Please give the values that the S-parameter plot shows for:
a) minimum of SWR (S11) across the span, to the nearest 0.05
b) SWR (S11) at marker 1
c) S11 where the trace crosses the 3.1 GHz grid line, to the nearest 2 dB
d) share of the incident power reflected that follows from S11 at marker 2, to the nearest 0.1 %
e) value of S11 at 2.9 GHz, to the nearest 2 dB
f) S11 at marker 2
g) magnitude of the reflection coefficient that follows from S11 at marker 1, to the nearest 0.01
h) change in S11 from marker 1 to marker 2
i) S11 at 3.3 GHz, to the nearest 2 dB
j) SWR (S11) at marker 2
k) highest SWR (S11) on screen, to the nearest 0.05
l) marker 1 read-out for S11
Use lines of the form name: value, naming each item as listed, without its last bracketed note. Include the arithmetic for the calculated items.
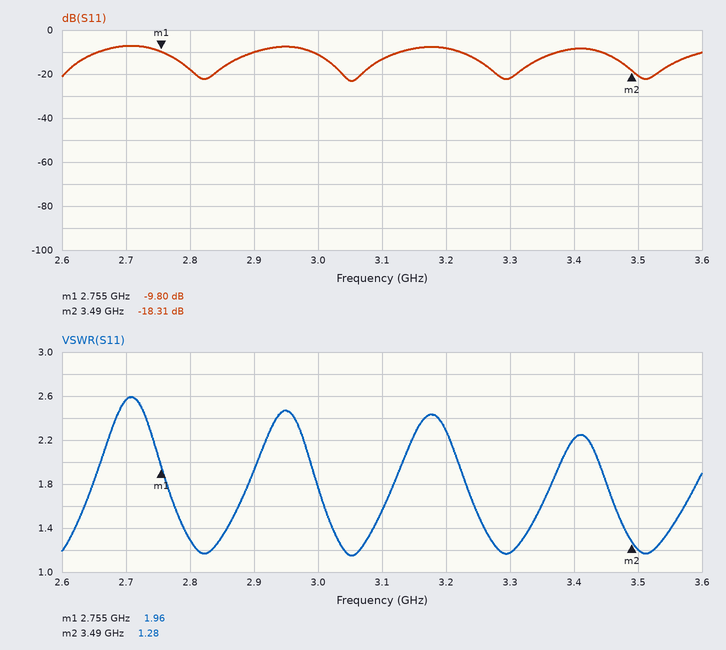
minimum of SWR (S11) across the span, to the nearest 0.05: 1.15
SWR (S11) at marker 1: 1.96
S11 where the trace crosses the 3.1 GHz grid line, to the nearest 2 dB: -14 dB
share of the incident power reflected that follows from S11 at marker 2, to the nearest 0.1 %: 10^(-18.31/10) ≈ 1.5 %
value of S11 at 2.9 GHz, to the nearest 2 dB: -10 dB
S11 at marker 2: -18.31 dB
magnitude of the reflection coefficient that follows from S11 at marker 1, to the nearest 0.01: 10^(-9.8/20) ≈ 0.32
change in S11 from marker 1 to marker 2: -18.31 − (-9.8) = -8.51 dB
S11 at 3.3 GHz, to the nearest 2 dB: -22 dB
SWR (S11) at marker 2: 1.28
highest SWR (S11) on screen, to the nearest 0.05: 2.60
marker 1 read-out for S11: -9.80 dB
